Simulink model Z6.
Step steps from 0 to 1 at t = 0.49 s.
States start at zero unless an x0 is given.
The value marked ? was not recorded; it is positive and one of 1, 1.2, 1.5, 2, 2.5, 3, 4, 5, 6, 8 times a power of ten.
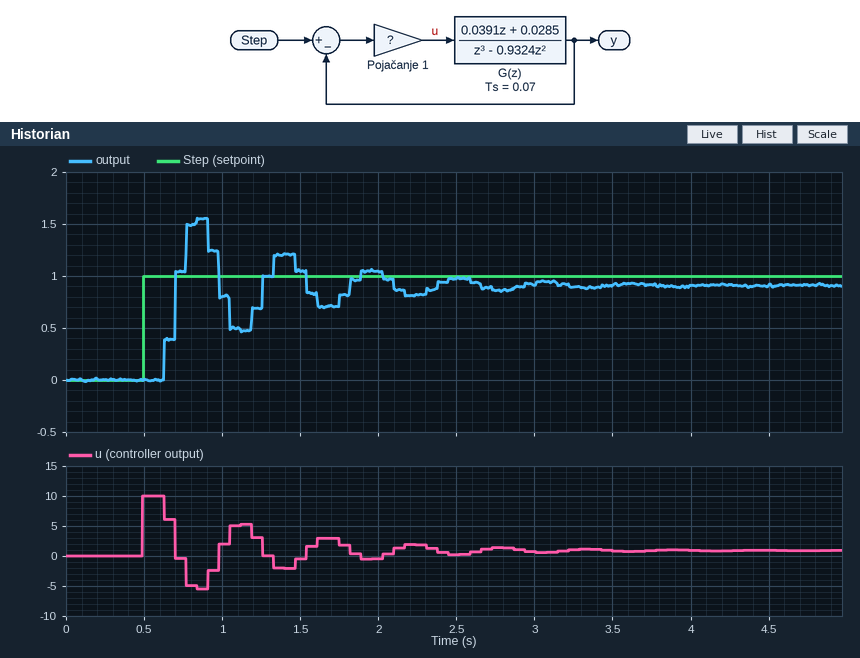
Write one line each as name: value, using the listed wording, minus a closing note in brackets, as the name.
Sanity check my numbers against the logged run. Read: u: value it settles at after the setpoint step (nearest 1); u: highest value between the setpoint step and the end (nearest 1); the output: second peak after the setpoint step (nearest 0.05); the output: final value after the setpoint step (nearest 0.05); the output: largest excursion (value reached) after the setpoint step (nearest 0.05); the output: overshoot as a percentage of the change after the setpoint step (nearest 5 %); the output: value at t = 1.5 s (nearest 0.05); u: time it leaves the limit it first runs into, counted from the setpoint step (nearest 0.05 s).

u: value it settles at after the setpoint step: 1
u: highest value between the setpoint step and the end: 10
the output: second peak after the setpoint step: 1.20
the output: final value after the setpoint step: 0.90
the output: largest excursion (value reached) after the setpoint step: 1.55
the output: overshoot as a percentage of the change after the setpoint step: 70 %
the output: value at t = 1.5 s: 1.05
u: time it leaves the limit it first runs into, counted from the setpoint step: 0.15 s
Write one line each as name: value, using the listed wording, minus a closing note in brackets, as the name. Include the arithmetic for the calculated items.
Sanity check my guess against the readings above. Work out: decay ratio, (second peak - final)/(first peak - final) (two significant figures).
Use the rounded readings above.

decay ratio, (second peak - final)/(first peak - final): (1.2 - 0.9) / (1.55 - 0.9) = 0.46
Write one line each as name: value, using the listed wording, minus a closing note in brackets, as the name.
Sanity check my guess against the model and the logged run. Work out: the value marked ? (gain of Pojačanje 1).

the value marked ?: 10
